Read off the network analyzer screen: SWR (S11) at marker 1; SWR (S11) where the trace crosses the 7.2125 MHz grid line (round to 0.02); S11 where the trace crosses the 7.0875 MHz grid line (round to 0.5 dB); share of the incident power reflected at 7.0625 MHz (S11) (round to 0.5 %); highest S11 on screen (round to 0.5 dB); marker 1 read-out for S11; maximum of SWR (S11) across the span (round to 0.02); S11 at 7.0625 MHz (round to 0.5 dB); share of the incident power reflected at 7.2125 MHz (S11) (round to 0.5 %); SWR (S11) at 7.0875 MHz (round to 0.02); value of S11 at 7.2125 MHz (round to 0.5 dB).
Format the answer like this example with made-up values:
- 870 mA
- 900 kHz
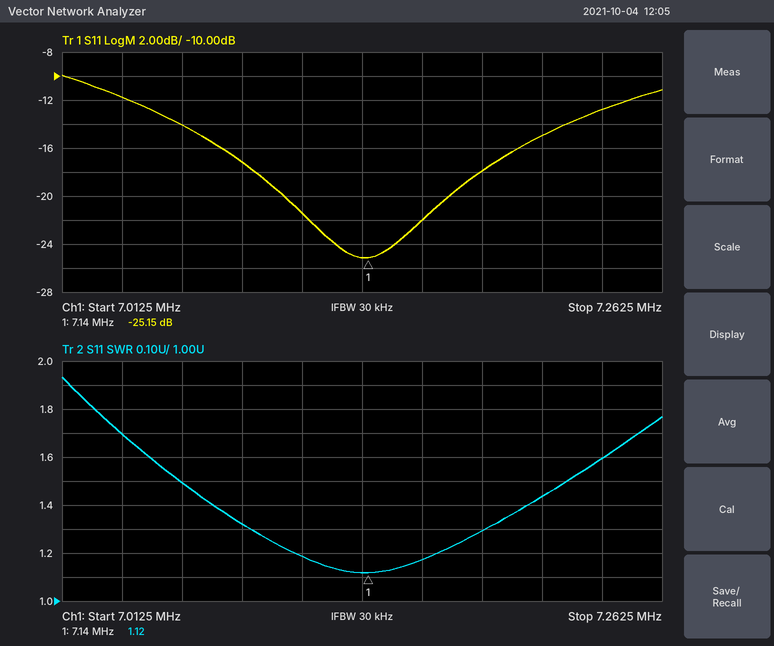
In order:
- 1.12
- 1.44
- -17.0 dB
- 4.0 %
- -10.0 dB
- -25.15 dB
- 1.94
- -14.0 dB
- 3.0 %
- 1.32
- -15.0 dB
